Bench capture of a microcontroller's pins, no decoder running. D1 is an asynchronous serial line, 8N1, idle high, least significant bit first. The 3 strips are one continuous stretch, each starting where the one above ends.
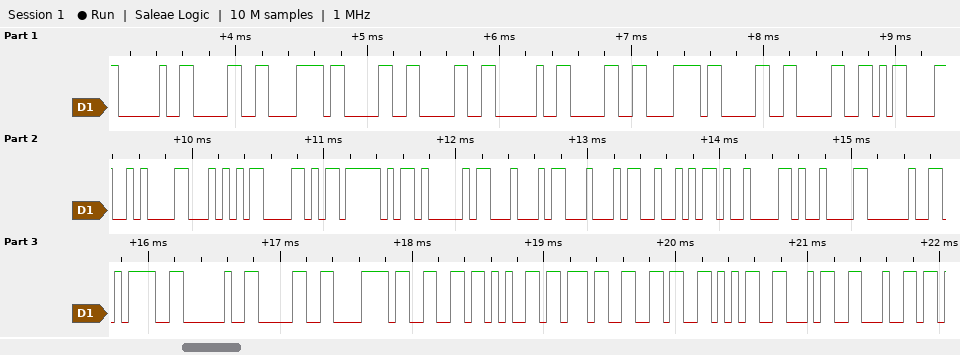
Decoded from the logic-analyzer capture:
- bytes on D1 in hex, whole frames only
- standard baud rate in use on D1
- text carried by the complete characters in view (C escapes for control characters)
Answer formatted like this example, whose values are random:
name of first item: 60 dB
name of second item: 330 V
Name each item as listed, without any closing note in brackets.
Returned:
bytes on D1 in hex, whole frames only: 20 30 78 30 30 20 30 78 30 30 0D 0A 54 58 5F 41 44 44 52 09 09 20 3D 20 30 78 66 65 37 36 35 34 64
standard baud rate in use on D1: 19200 baud
text carried by the complete characters in view: " 0x00 0x00\r\nTX_ADDR\t\t = 0xfe7654d"
